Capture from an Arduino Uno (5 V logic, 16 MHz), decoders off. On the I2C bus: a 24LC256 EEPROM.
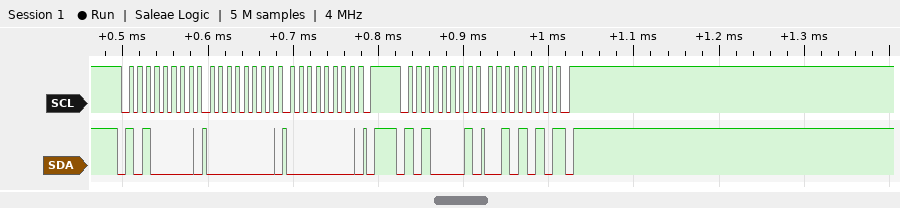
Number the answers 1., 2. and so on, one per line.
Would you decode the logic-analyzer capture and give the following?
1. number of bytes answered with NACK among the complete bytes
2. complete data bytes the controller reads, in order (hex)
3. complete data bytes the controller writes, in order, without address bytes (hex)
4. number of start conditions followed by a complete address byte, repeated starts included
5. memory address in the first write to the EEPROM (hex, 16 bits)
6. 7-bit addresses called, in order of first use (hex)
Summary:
1. 1
2. 2A
3. 00 00
4. 2
5. 0x0000
6. 0x50
